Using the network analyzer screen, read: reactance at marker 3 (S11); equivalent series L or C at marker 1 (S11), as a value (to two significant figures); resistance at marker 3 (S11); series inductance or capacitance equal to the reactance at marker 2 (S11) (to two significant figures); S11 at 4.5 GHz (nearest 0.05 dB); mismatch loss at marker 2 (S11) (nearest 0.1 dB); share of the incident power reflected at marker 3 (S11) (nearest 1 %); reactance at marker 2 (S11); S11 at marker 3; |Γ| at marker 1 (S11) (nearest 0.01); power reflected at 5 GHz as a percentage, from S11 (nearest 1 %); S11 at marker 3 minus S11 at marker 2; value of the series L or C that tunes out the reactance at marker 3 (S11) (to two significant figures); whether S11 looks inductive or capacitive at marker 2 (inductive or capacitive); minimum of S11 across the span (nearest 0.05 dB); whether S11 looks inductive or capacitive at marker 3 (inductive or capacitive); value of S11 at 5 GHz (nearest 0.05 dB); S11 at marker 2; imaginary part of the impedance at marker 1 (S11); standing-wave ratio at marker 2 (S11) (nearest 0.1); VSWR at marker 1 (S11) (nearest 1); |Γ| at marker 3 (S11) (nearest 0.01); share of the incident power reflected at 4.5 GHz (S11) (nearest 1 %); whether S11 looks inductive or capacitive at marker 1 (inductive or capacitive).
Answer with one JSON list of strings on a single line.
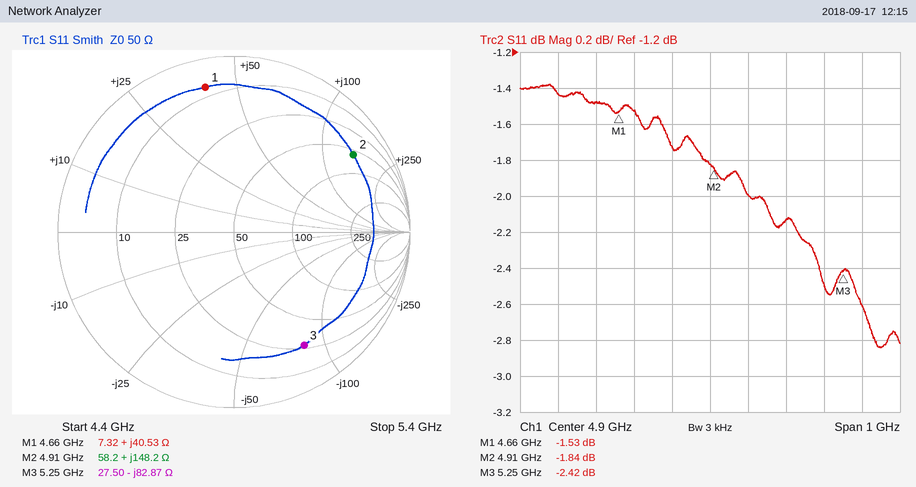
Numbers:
["-82.87 Ω", "1.4 nH", "27.50 Ω", "4.8 nH", "-1.45 dB", "4.6 dB", "57 %", "+148.2 Ω", "-2.42 dB", "0.84", "63 %", "-0.58 dB", "2.5 nH", "inductive", "-2.85 dB", "capacitive", "-2.00 dB", "-1.84 dB", "+40.53 Ω", "9.5", "11", "0.76", "72 %", "inductive"]
